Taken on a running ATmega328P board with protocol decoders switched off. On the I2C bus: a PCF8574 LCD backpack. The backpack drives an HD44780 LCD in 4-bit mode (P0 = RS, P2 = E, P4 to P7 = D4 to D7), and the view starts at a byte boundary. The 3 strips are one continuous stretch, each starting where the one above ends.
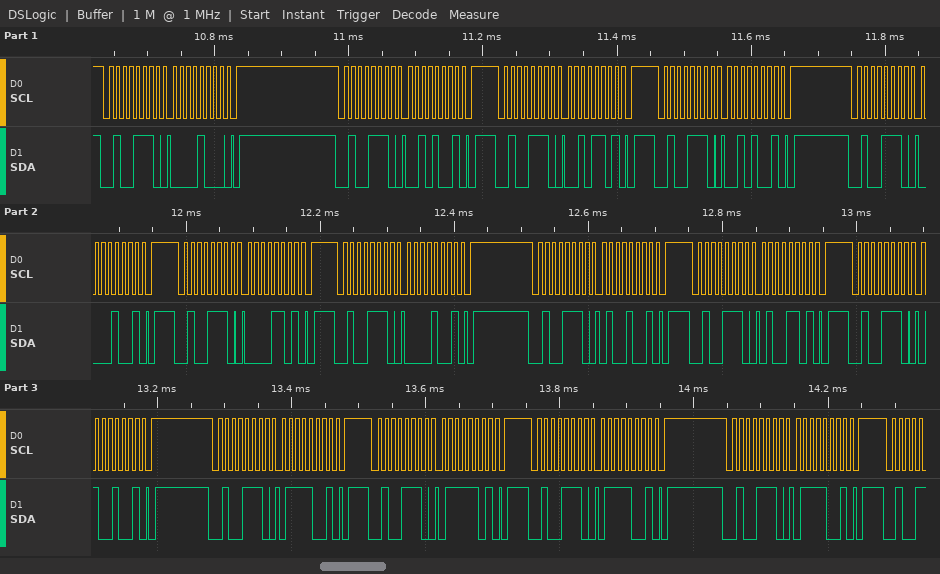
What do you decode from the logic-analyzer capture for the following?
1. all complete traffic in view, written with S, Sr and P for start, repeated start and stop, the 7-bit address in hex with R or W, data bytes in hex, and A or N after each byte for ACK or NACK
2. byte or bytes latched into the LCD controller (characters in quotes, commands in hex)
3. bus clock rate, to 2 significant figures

S 27W A 08 A P S 27W A 29 A P S 27W A 2D A P S 27W A 29 A P S 27W A 09 A P S 27W A 0D A P S 27W A 09 A P S 27W A 49 A P S 27W A 4D A P S 27W A 49 A P S 27W A 79 A P S 27W A 7D A P S 27W A 79 A P S 27W A 79 A P
' ' 'G'
100 kHz
